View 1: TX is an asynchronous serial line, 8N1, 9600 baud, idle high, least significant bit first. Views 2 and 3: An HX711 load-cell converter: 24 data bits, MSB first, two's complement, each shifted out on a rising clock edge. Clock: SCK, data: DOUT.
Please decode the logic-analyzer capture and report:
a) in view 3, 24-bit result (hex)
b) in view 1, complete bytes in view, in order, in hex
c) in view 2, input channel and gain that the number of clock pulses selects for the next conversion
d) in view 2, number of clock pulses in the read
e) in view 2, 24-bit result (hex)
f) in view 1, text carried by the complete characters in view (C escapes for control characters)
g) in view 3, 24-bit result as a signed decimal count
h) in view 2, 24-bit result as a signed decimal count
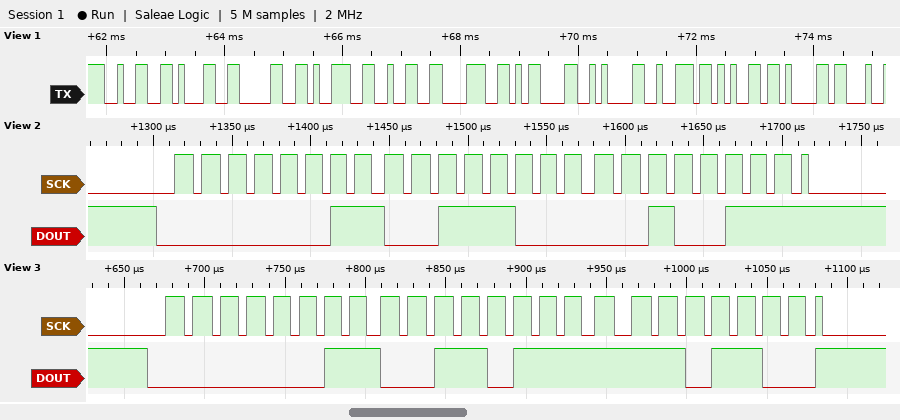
0x0337EC
32 31 30 39 32 38 0D 0A 72 65 61
channel A, gain 128
25
0x033827
"210928\r\nrea"
210924
210983
